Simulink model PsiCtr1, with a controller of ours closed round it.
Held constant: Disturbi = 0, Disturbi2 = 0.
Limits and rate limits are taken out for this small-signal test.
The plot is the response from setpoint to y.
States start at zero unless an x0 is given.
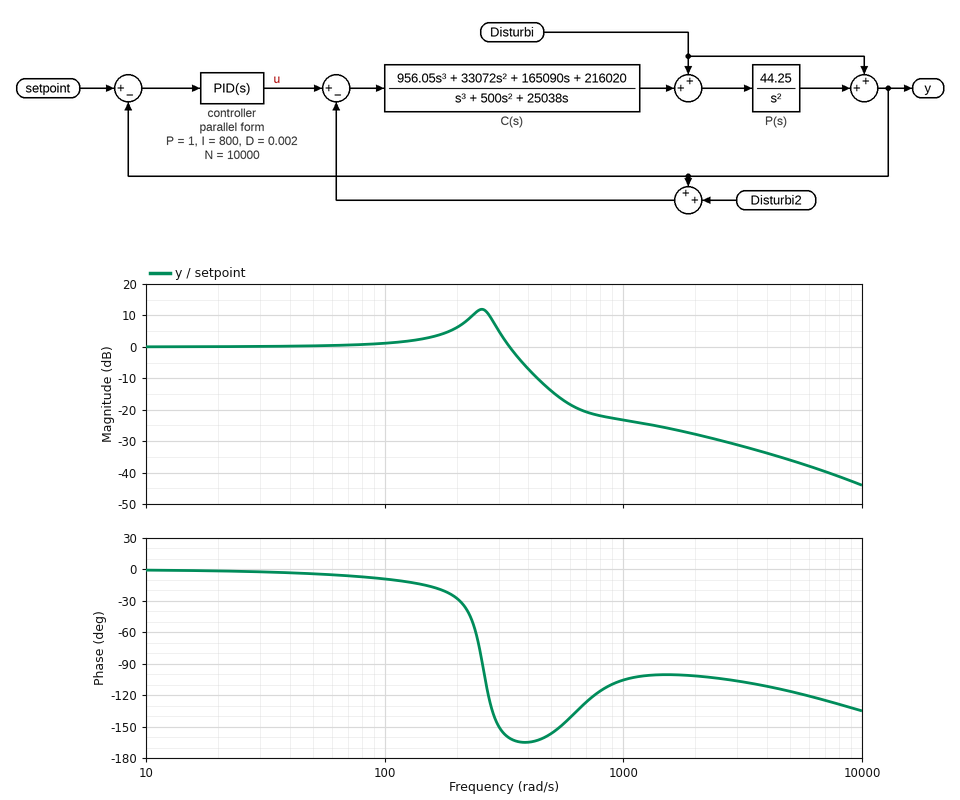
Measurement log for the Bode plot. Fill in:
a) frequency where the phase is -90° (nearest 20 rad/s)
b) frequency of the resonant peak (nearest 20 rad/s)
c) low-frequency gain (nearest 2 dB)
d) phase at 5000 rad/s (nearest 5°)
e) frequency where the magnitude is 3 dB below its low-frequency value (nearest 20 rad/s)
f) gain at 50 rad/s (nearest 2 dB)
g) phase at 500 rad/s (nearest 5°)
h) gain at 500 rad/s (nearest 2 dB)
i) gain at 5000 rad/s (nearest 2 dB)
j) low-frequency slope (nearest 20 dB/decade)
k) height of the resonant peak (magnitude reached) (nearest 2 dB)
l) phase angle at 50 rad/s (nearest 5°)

260 rad/s
260 rad/s
0 dB
-115°
360 rad/s
0 dB
-155°
-14 dB
-36 dB
0 dB/decade
12 dB
-5°
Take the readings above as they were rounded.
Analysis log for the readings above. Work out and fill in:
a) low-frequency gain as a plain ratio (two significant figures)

1.0
